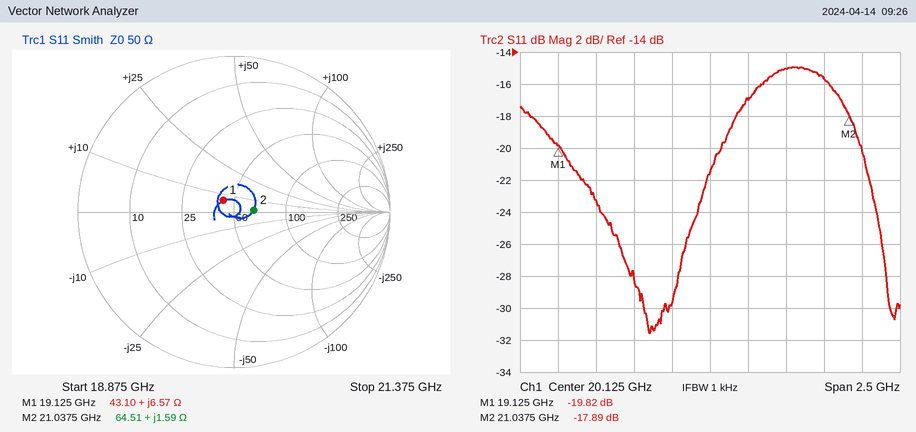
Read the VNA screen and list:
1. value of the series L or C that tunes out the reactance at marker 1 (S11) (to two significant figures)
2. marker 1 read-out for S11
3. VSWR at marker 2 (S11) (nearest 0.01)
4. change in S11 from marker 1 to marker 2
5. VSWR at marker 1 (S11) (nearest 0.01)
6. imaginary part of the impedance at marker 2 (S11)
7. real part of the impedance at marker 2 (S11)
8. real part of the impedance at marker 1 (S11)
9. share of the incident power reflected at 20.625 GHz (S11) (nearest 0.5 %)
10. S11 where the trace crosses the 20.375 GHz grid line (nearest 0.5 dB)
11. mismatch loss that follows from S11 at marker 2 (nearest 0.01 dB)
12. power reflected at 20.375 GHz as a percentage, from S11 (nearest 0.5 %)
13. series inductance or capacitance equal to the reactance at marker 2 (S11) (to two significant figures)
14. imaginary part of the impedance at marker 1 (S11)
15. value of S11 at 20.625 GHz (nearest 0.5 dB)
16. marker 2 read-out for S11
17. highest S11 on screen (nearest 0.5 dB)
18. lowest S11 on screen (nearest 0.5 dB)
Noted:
1.3 pF
-19.82 dB
1.29
1.93 dB
1.23
+1.59 Ω
64.51 Ω
43.10 Ω
3.0 %
-17.0 dB
0.07 dB
2.0 %
12 pH
+6.57 Ω
-15.0 dB
-17.89 dB
-15.0 dB
-31.5 dB
